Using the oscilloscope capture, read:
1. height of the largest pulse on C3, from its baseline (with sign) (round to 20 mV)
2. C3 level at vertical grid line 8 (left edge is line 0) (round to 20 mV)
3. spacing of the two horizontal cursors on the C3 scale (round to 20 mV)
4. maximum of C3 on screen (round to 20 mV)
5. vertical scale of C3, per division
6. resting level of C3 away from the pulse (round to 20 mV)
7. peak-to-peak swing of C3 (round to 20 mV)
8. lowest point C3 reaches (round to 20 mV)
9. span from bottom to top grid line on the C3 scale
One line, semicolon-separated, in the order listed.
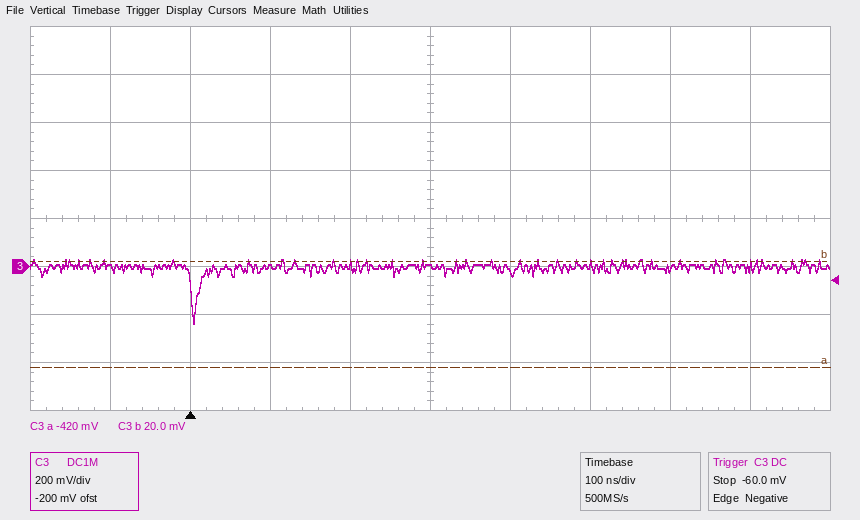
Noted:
-240 mV; 0 mV; 440 mV; 20 mV; 200 mV; 0 mV; 260 mV; -240 mV; 1.6 V
